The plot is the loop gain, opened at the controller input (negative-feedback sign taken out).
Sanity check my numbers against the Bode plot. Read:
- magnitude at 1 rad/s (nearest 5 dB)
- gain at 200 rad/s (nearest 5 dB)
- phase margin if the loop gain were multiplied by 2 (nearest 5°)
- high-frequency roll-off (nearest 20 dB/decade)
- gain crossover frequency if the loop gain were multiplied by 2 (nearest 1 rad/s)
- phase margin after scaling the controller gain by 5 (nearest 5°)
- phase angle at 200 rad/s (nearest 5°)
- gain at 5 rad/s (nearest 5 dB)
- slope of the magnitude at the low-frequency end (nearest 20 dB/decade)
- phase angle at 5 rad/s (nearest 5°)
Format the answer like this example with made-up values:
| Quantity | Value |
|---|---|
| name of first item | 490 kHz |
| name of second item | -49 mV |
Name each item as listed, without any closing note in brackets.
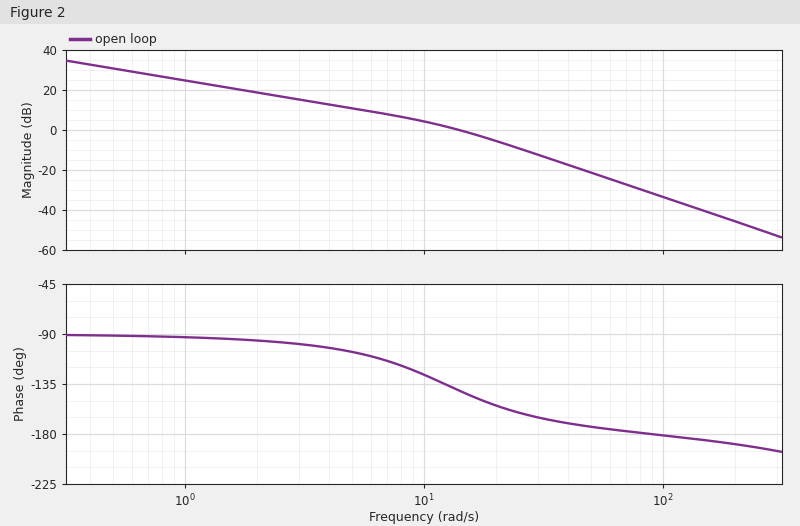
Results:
| Quantity | Value |
|---|---|
| magnitude at 1 rad/s | 25 dB |
| gain at 200 rad/s | -45 dB |
| phase margin if the loop gain were multiplied by 2 | 25° |
| high-frequency roll-off | -40 dB/decade |
| gain crossover frequency if the loop gain were multiplied by 2 | 21 rad/s |
| phase margin after scaling the controller gain by 5 | 15° |
| phase angle at 200 rad/s | -190° |
| gain at 5 rad/s | 10 dB |
| slope of the magnitude at the low-frequency end | -20 dB/decade |
| phase angle at 5 rad/s | -105° |
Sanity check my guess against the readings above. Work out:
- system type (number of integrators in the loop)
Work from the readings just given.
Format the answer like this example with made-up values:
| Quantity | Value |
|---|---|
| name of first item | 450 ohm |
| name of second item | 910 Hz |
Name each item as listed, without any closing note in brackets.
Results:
| Quantity | Value |
|---|---|
| system type | 1 |
